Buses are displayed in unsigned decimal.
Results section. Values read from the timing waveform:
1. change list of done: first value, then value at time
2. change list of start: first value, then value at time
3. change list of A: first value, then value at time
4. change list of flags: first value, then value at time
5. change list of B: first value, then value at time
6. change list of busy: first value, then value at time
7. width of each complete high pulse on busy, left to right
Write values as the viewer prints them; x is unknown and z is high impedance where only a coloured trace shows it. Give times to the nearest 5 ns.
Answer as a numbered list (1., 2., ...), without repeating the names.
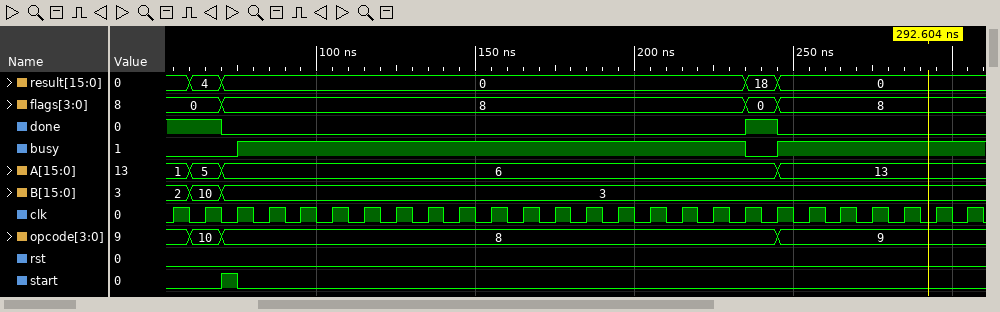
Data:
1. 1, 0 at 70 ns, 1 at 235 ns, 0 at 245 ns
2. 0, 1 at 70 ns, 0 at 75 ns
3. 1, 5 at 60 ns, 6 at 70 ns, 13 at 245 ns
4. 0, 8 at 70 ns, 0 at 235 ns, 8 at 245 ns
5. 2, 10 at 60 ns, 3 at 70 ns
6. 0, 1 at 75 ns, 0 at 235 ns, 1 at 245 ns
7. 160 ns
